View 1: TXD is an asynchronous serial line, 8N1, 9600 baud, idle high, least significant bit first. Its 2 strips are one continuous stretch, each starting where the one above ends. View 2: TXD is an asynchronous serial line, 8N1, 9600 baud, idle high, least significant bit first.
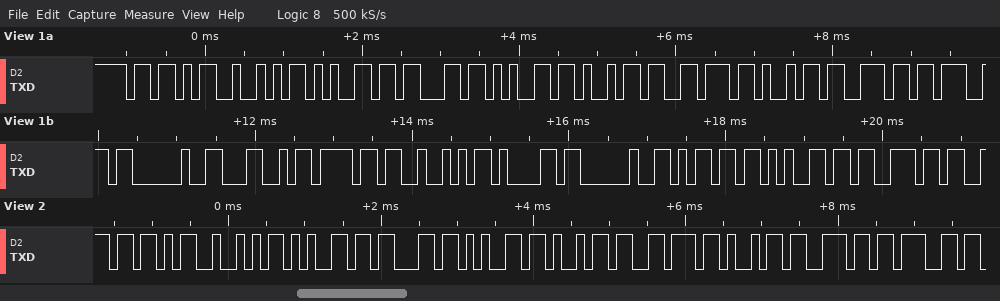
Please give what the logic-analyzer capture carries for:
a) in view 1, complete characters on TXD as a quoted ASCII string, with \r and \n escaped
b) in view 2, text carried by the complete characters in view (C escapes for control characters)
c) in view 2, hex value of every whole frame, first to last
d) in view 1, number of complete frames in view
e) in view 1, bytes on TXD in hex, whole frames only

"[Receiving LoRa mes"
"[Receiving"
5B 52 65 63 65 69 76 69 6E 67
19
0x5B 0x52 0x65 0x63 0x65 0x69 0x76 0x69 0x6E 0x67 0x20 0x4C 0x6F 0x52 0x61 0x20 0x6D 0x65 0x73
